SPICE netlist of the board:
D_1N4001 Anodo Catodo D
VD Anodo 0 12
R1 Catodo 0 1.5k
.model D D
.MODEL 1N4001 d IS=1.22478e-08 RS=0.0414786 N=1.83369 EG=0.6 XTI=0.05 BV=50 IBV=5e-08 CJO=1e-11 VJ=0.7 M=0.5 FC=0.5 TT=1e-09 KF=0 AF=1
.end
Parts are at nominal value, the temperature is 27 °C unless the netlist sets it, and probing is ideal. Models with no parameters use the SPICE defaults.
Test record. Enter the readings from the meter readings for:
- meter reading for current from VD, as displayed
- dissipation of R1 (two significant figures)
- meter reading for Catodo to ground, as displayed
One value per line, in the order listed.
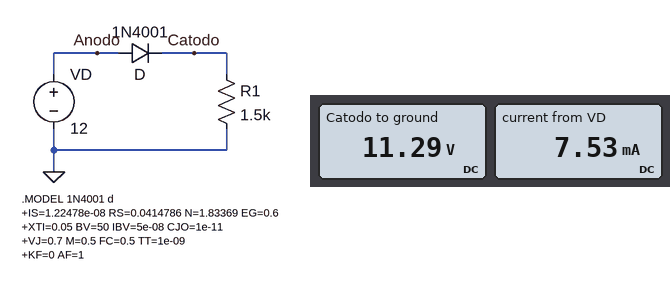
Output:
7.53 mA
85 mW
11.29 V
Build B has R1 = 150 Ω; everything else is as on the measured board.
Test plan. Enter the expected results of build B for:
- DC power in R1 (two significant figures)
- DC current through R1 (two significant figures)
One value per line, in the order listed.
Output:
840 mW
75 mA
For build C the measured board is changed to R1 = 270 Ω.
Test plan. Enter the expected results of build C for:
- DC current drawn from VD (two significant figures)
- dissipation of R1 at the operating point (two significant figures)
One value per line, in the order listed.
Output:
42 mA
470 mW
